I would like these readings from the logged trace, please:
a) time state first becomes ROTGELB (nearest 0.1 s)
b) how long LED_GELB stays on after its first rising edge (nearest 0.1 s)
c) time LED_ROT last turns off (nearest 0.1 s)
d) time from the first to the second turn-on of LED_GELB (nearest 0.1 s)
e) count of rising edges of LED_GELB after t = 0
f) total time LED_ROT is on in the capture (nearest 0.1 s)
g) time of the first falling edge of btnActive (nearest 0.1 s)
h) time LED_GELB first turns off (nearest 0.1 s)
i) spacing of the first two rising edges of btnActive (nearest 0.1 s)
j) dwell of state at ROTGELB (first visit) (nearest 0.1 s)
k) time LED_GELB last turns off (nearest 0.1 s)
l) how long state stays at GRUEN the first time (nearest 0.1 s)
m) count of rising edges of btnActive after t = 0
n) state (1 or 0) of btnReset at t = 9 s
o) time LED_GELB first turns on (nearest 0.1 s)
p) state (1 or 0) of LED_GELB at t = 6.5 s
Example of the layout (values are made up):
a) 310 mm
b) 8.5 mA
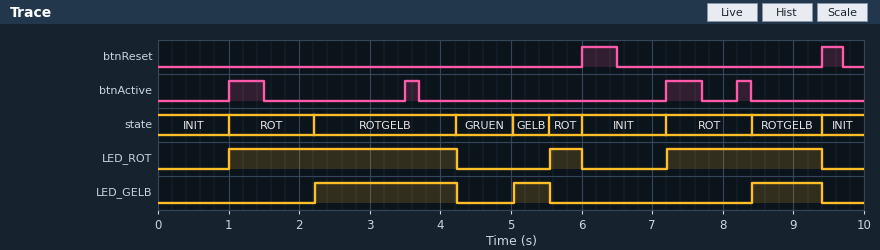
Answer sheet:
a) 2.2 s
b) 2.0 s
c) 9.4 s
d) 2.8 s
e) 3
f) 5.9 s
g) 1.5 s
h) 4.2 s
i) 2.5 s
j) 2.0 s
k) 9.4 s
l) 0.8 s
m) 4
n) 0
o) 2.2 s
p) 0
